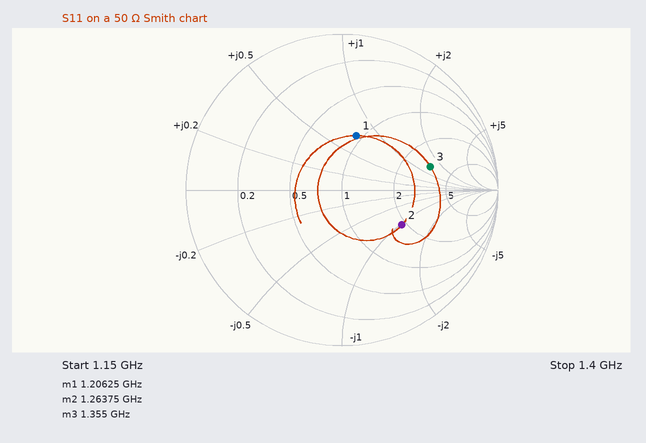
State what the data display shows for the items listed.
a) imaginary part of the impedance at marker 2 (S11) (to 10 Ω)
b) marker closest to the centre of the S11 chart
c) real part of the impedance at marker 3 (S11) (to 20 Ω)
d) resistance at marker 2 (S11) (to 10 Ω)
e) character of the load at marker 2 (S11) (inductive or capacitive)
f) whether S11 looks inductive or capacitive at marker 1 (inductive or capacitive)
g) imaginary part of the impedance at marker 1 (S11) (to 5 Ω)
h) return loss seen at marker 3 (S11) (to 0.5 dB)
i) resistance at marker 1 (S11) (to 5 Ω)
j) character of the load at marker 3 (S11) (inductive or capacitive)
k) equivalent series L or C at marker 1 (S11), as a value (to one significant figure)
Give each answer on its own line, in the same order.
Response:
-50 Ω
marker 1
160 Ω
90 Ω
capacitive
inductive
+35 Ω
4.5 dB
45 Ω
inductive
5 nH
